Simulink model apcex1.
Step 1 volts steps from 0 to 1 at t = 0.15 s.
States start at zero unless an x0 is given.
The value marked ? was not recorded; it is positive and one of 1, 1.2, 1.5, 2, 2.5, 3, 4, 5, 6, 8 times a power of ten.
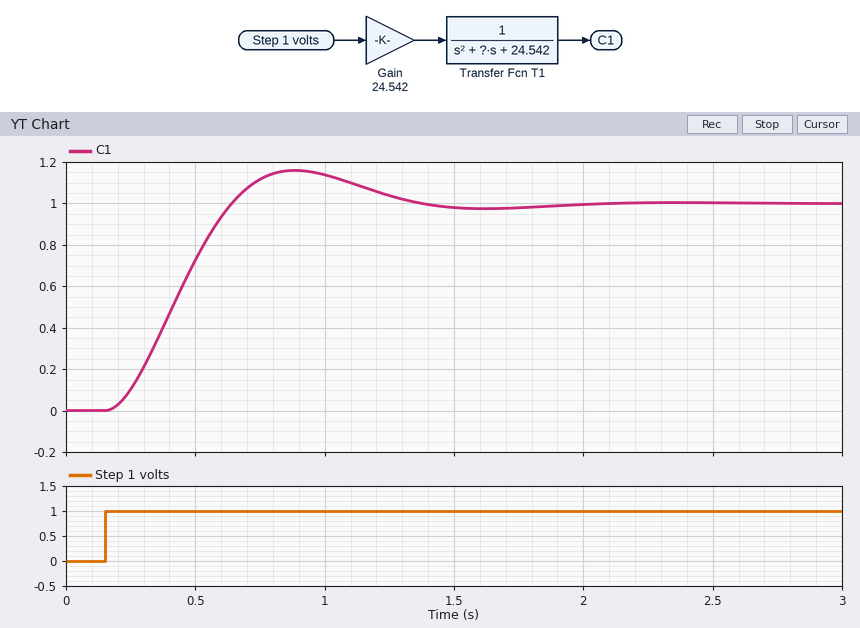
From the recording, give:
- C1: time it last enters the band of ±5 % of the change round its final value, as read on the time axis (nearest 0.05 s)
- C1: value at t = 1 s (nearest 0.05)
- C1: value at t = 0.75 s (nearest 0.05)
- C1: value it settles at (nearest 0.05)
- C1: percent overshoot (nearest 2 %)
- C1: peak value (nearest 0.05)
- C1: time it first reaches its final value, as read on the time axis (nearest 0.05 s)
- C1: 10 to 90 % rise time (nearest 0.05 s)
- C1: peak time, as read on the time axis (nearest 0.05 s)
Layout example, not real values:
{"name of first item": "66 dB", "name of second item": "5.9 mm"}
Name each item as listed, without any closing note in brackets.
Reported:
{"C1: time it last enters the band of ±5 % of the change round its final value, as read on the time axis": "1.20 s", "C1: value at t = 1 s": "1.15", "C1: value at t = 0.75 s": "1.10", "C1: value it settles at": "1.00", "C1: percent overshoot": "16 %", "C1: peak value": "1.15", "C1: time it first reaches its final value, as read on the time axis": "0.65 s", "C1: 10 to 90 % rise time": "0.35 s", "C1: peak time, as read on the time axis": "0.90 s"}
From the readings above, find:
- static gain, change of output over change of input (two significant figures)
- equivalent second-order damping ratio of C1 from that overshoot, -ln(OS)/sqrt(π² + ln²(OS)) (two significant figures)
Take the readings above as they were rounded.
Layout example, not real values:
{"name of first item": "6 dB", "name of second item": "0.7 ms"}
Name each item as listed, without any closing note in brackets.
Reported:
{"static gain, change of output over change of input": "1.0", "equivalent second-order damping ratio of C1 from that overshoot, -ln(OS)/sqrt(π² + ln²(OS))": "0.50"}
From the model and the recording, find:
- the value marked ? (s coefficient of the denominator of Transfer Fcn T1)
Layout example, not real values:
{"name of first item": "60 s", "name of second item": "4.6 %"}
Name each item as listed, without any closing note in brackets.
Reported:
{"the value marked ?": "5"}
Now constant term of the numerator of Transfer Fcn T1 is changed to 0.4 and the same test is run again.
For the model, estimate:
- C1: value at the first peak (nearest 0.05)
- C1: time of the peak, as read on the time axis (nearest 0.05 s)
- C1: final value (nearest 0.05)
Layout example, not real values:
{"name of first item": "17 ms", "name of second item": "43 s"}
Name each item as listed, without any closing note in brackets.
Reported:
{"C1: value at the first peak": "0.45", "C1: time of the peak, as read on the time axis": "0.90 s", "C1: final value": "0.40"}
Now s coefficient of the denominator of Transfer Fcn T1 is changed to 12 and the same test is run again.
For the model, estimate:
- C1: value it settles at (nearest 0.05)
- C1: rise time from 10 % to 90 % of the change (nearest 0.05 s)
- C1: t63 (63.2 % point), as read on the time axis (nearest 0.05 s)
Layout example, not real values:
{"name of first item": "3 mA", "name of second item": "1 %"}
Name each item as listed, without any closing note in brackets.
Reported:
{"C1: value it settles at": "1.00", "C1: rise time from 10 % to 90 % of the change": "0.90 s", "C1: t63 (63.2 % point), as read on the time axis": "0.65 s"}
